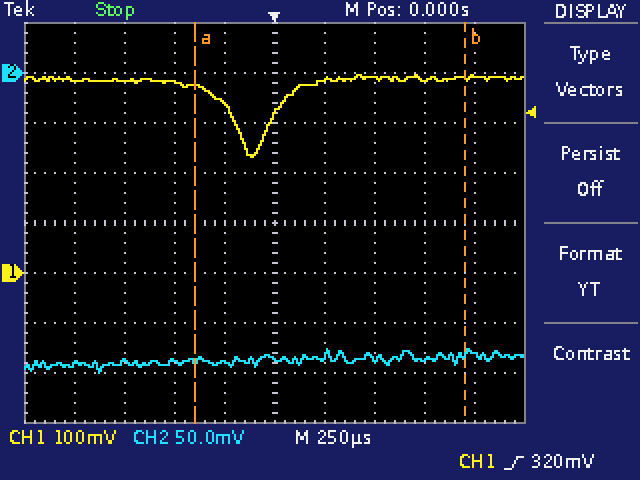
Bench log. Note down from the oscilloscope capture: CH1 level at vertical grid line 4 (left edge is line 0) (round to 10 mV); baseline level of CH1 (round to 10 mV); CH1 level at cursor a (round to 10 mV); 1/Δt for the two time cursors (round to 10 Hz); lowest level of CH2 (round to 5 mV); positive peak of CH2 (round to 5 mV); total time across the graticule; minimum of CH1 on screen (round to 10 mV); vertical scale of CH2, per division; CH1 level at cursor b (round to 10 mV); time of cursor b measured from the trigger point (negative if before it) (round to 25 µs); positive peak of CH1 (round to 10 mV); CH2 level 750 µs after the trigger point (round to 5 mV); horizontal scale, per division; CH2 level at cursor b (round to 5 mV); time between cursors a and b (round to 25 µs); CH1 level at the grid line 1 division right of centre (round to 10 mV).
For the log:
340 mV
390 mV
370 mV
740 Hz
-300 mV
-275 mV
2.5 ms
230 mV
50 mV
390 mV
+950 µs
400 mV
-285 mV
250 µs
-280 mV
1.350 ms
390 mV
